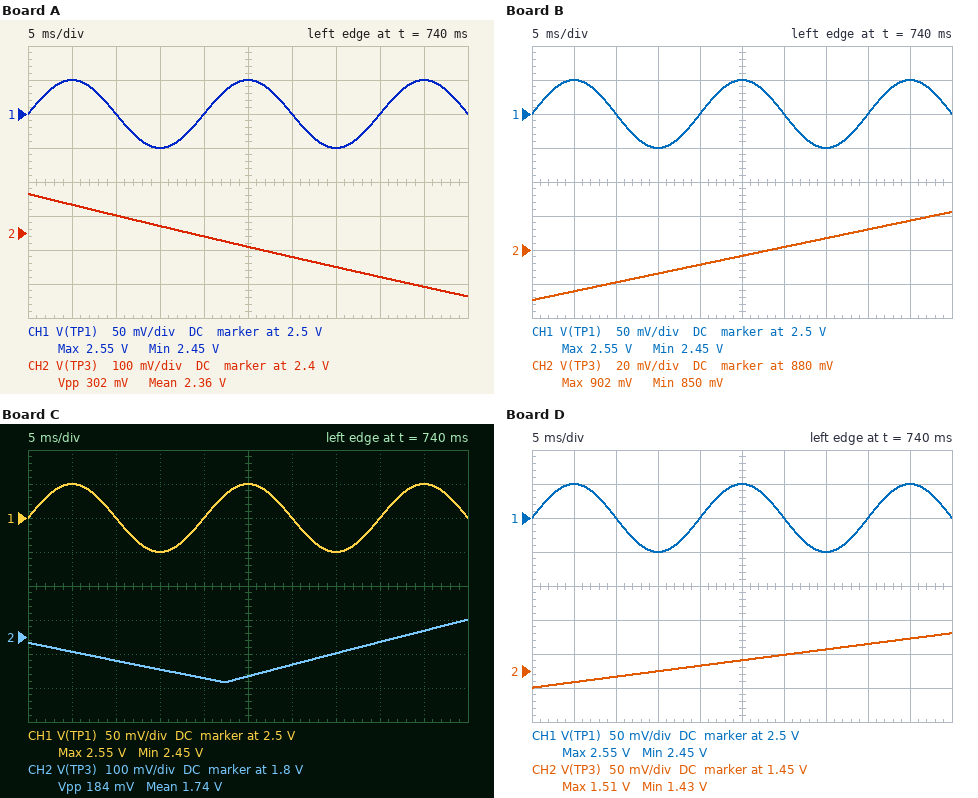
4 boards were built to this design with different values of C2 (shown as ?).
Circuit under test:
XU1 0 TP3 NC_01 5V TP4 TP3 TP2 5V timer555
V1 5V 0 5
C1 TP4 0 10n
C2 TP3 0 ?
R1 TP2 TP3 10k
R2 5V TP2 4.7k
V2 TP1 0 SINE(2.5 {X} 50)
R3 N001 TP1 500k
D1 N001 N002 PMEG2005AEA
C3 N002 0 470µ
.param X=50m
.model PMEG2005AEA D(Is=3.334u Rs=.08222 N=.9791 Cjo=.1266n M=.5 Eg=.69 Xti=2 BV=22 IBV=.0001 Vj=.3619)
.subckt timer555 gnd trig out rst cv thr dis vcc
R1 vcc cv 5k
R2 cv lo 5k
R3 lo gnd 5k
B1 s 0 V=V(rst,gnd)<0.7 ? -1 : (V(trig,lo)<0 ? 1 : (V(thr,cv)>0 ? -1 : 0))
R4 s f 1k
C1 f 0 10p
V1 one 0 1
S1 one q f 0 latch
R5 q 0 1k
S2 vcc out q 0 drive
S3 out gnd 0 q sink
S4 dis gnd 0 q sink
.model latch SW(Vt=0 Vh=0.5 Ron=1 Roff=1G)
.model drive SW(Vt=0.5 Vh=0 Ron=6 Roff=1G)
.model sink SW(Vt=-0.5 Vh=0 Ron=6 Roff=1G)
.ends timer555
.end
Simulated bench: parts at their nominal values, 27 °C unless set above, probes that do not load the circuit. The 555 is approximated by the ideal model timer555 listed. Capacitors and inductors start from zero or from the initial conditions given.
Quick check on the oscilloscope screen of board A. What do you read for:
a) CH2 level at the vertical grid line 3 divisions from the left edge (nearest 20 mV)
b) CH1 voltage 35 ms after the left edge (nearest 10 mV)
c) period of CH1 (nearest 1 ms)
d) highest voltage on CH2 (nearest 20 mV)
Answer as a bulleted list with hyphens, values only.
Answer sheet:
- 2.42 V
- 2.45 V
- 20 ms
- 2.52 V
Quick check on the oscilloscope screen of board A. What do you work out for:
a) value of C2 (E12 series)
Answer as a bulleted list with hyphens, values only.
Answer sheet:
- 39 µF
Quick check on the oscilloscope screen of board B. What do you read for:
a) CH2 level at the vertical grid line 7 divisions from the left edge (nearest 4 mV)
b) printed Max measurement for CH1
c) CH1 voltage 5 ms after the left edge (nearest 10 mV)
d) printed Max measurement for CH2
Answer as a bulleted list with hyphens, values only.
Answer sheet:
- 888 mV
- 2.55 V
- 2.55 V
- 902 mV
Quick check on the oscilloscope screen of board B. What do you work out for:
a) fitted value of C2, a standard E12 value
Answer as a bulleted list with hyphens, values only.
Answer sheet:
- 270 µF
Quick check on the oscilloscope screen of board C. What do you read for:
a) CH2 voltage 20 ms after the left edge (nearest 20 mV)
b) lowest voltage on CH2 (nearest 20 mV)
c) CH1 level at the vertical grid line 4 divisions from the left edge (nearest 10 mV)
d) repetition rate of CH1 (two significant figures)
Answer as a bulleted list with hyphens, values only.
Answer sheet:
- 1.68 V
- 1.66 V
- 2.50 V
- 50 Hz
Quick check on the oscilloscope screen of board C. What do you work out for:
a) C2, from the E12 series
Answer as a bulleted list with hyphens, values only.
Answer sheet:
- 33 µF
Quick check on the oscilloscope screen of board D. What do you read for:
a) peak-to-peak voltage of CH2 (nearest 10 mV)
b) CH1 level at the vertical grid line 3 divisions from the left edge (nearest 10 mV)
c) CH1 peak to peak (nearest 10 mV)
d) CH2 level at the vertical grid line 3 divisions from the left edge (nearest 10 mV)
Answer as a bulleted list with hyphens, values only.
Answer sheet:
- 80 mV
- 2.45 V
- 100 mV
- 1.45 V
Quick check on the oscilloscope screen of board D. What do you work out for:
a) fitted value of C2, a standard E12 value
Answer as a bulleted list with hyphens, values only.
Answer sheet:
- 150 µF
